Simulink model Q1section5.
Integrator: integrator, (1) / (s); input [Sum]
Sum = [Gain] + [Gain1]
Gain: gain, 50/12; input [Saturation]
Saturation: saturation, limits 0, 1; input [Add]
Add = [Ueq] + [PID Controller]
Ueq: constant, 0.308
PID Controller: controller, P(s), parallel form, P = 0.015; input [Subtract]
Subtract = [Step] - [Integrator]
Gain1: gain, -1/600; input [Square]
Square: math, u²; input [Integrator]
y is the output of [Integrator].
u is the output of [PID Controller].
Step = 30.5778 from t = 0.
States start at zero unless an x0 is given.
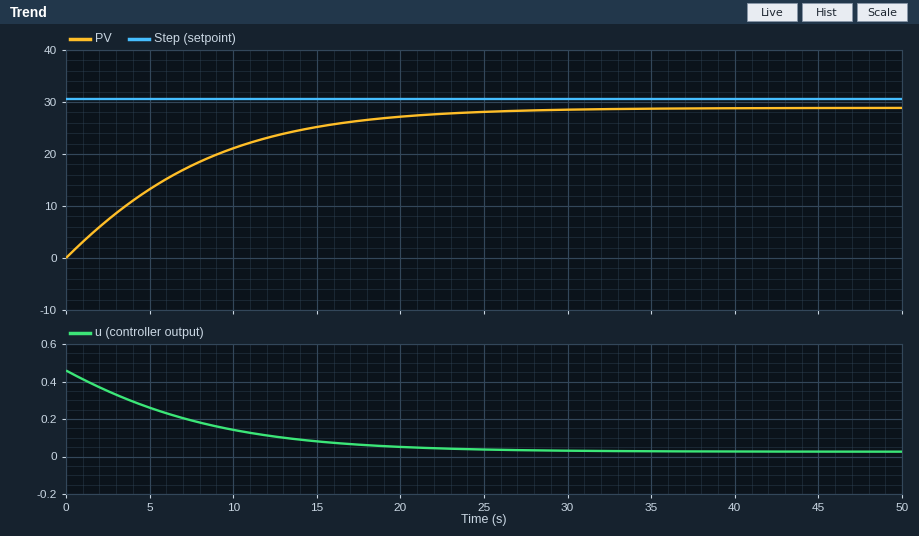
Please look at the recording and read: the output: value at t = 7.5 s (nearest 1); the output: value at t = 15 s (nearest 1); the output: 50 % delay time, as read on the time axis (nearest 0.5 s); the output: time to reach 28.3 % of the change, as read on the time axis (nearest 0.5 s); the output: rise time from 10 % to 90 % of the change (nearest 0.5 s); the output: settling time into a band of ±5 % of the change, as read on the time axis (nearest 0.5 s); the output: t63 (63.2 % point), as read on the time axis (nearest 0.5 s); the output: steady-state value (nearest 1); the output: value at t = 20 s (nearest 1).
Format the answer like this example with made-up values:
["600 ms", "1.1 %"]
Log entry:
["18", "25", "5.5 s", "3.0 s", "15.5 s", "21.0 s", "8.0 s", "29", "27"]
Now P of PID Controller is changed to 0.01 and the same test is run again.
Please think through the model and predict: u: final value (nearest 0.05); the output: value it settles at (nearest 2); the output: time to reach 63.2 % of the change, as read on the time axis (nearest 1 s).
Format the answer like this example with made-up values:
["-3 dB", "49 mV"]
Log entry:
["0.00", "28", "9 s"]
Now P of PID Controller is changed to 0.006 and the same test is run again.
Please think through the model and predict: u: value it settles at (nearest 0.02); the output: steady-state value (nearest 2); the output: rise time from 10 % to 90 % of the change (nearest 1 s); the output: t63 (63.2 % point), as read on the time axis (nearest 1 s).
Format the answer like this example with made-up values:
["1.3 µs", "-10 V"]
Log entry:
["0.02", "28", "22 s", "11 s"]
